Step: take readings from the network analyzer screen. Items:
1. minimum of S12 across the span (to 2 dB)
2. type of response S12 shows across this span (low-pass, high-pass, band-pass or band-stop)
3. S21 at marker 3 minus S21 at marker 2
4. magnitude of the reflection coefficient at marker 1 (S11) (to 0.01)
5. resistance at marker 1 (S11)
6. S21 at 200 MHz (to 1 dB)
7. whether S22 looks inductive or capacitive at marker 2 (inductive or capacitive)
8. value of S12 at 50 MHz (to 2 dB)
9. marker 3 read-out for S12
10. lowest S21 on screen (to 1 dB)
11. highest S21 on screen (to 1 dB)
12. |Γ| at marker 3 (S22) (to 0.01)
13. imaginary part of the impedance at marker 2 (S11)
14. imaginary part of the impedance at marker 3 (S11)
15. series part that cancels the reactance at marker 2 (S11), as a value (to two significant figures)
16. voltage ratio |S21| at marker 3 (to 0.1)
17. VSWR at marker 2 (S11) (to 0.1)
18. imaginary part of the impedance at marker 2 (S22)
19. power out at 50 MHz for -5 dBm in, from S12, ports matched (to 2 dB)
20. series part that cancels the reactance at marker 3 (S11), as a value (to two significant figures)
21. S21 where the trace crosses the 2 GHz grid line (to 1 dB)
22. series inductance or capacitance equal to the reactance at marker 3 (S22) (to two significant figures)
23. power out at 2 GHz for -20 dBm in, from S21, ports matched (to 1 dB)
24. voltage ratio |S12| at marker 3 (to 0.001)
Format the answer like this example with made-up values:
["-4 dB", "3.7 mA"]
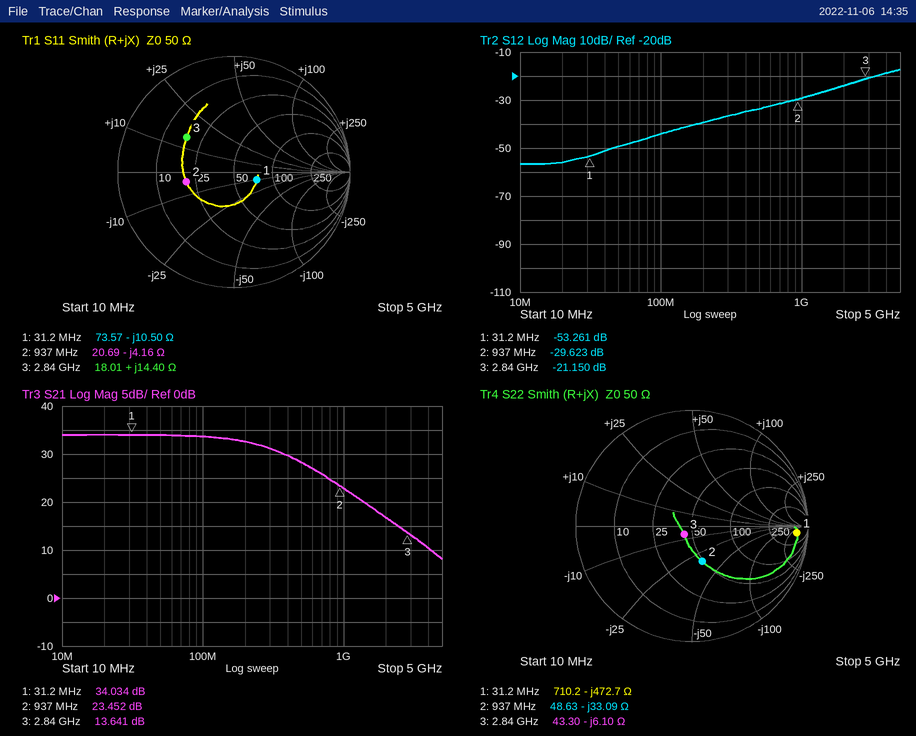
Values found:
["-56 dB", "high-pass", "-9.811 dB", "0.21", "73.57 Ω", "33 dB", "capacitive", "-50 dB", "-21.150 dB", "8 dB", "34 dB", "0.10", "-4.16 Ω", "+14.40 Ω", "710 pH", "4.8", "2.4", "-33.09 Ω", "-54 dBm", "3.9 pF", "17 dB", "9.2 pF", "-3 dBm", "0.088"]
